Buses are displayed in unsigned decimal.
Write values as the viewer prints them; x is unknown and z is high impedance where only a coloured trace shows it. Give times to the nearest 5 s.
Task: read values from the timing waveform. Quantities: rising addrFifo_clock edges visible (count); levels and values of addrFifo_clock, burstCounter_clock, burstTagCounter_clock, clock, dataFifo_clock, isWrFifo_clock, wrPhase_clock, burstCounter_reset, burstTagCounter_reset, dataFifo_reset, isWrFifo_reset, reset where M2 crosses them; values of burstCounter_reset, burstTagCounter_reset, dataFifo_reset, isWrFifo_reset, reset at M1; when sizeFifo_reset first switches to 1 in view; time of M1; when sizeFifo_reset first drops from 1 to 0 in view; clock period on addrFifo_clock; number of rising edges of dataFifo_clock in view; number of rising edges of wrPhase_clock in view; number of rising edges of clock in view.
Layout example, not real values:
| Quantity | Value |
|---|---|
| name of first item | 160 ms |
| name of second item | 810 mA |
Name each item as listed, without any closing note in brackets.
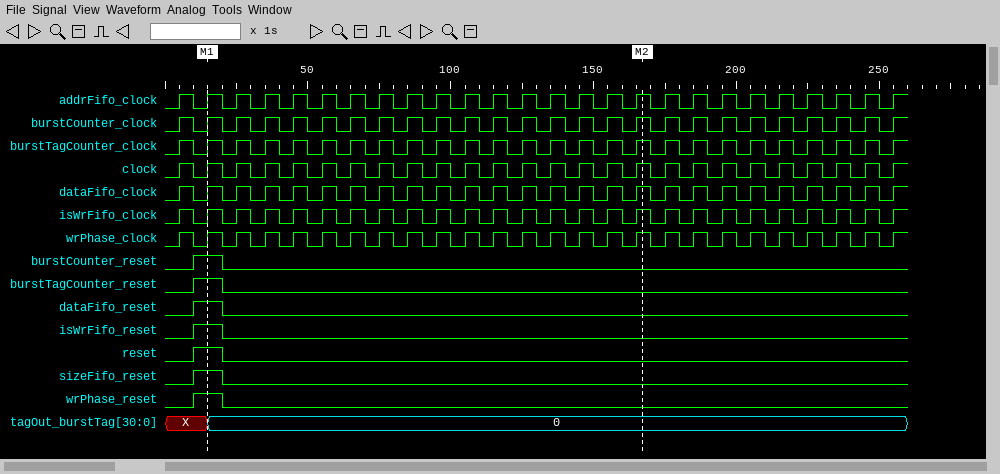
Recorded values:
| Quantity | Value |
|---|---|
| rising addrFifo_clock edges visible | 26 |
| levels and values of addrFifo_clock, burstCounter_clock, burstTagCounter_clock, clock, dataFifo_clock, isWrFifo_clock, wrPhase_clock, burstCounter_reset, burstTagCounter_reset, dataFifo_reset, isWrFifo_reset, reset where M2 crosses them | addrFifo_clock=1, burstCounter_clock=1, burstTagCounter_clock=1, clock=1, dataFifo_clock=1, isWrFifo_clock=1, wrPhase_clock=1, burstCounter_reset=0, burstTagCounter_reset=0, dataFifo_reset=0, isWrFifo_reset=0, reset=0 |
| values of burstCounter_reset, burstTagCounter_reset, dataFifo_reset, isWrFifo_reset, reset at M1 | burstCounter_reset=1, burstTagCounter_reset=1, dataFifo_reset=1, isWrFifo_reset=1, reset=1 |
| when sizeFifo_reset first switches to 1 in view | 10 s |
| time of M1 | 15 s |
| when sizeFifo_reset first drops from 1 to 0 in view | 20 s |
| clock period on addrFifo_clock | 10 s |
| number of rising edges of dataFifo_clock in view | 26 |
| number of rising edges of wrPhase_clock in view | 26 |
| number of rising edges of clock in view | 26 |
